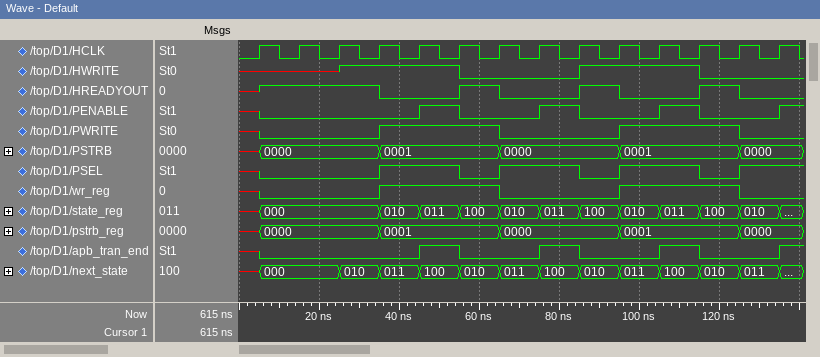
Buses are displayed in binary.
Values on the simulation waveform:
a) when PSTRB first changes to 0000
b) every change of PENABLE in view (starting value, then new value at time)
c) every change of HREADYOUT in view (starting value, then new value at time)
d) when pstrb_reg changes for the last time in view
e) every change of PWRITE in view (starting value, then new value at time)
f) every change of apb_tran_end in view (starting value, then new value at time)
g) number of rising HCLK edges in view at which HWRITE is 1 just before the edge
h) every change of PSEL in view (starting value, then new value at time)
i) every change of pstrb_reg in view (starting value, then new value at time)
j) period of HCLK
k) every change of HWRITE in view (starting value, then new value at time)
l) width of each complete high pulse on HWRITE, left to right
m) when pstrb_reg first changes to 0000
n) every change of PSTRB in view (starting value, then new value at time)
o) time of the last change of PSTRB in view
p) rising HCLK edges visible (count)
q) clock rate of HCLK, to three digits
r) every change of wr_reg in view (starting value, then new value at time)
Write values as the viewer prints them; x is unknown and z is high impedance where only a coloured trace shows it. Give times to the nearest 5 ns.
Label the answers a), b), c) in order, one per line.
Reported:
a) 5 ns
b) x, 0 at 5 ns, 1 at 45 ns, 0 at 55 ns, 1 at 75 ns, 0 at 85 ns, 1 at 105 ns, 0 at 115 ns, 1 at 135 ns
c) x, 1 at 5 ns, 0 at 35 ns, 1 at 55 ns, 0 at 65 ns, 1 at 85 ns, 0 at 95 ns, 1 at 115 ns, 0 at 125 ns
d) 125 ns
e) x, 0 at 5 ns, 1 at 35 ns, 0 at 65 ns, 1 at 95 ns, 0 at 125 ns
f) x, 0 at 5 ns, 1 at 45 ns, 0 at 55 ns, 1 at 75 ns, 0 at 85 ns, 1 at 105 ns, 0 at 115 ns, 1 at 135 ns
g) 6
h) x, 0 at 5 ns, 1 at 35 ns, 0 at 55 ns, 1 at 65 ns, 0 at 85 ns, 1 at 95 ns, 0 at 115 ns, 1 at 125 ns
i) x, 0000 at 5 ns, 0001 at 35 ns, 0000 at 65 ns, 0001 at 95 ns, 0000 at 125 ns
j) 10 ns
k) x, 1 at 25 ns, 0 at 55 ns, 1 at 85 ns, 0 at 115 ns
l) 30 ns
m) 5 ns
n) x, 0000 at 5 ns, 0001 at 35 ns, 0000 at 65 ns, 0001 at 95 ns, 0000 at 125 ns
o) 125 ns
p) 14
q) 100 MHz
r) x, 0 at 5 ns, 1 at 35 ns, 0 at 65 ns, 1 at 95 ns, 0 at 125 ns
